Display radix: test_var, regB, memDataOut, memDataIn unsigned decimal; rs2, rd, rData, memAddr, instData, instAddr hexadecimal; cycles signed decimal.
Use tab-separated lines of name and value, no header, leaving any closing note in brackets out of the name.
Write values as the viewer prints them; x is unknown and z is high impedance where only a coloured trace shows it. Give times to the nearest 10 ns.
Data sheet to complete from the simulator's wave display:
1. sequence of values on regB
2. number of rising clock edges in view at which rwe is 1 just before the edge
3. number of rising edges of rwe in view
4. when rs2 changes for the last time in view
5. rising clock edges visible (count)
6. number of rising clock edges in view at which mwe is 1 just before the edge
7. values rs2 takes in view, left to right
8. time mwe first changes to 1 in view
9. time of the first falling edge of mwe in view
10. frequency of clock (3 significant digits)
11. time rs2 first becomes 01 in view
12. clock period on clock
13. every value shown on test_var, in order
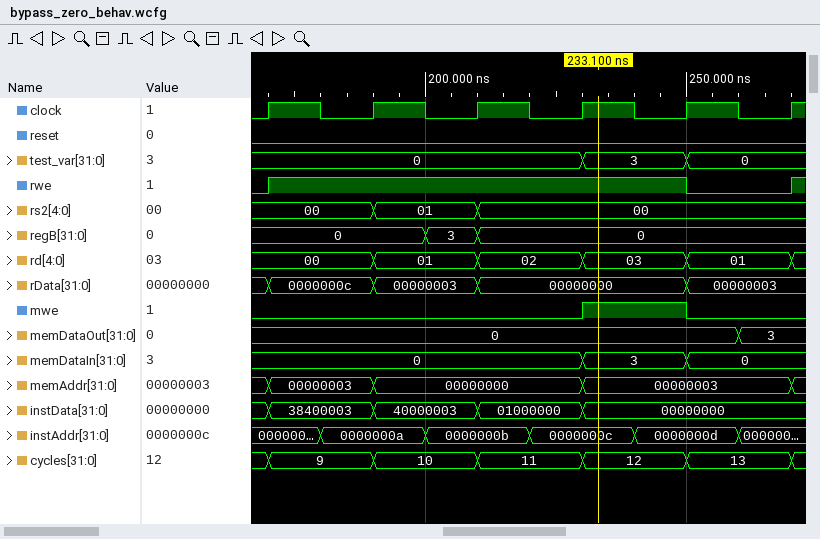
sequence of values on regB	0, 3, 0
number of rising clock edges in view at which rwe is 1 just before the edge	4
number of rising edges of rwe in view	2
when rs2 changes for the last time in view	210 ns
rising clock edges visible	6
number of rising clock edges in view at which mwe is 1 just before the edge	1
values rs2 takes in view, left to right	00, 01, 00
time mwe first changes to 1 in view	230 ns
time of the first falling edge of mwe in view	250 ns
frequency of clock	50.0 MHz
time rs2 first becomes 01 in view	190 ns
clock period on clock	20 ns
every value shown on test_var, in order	0, 3, 0
